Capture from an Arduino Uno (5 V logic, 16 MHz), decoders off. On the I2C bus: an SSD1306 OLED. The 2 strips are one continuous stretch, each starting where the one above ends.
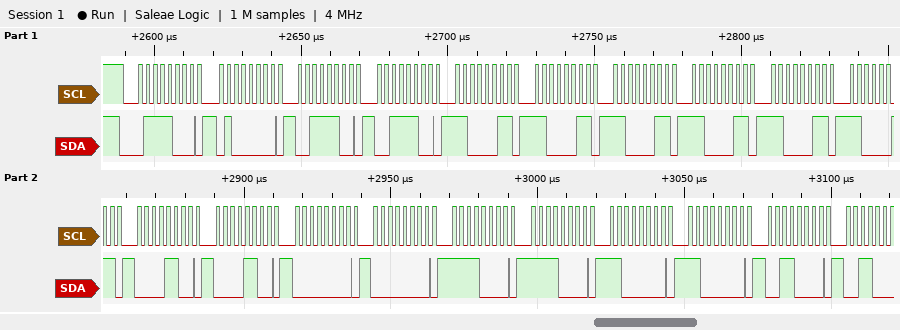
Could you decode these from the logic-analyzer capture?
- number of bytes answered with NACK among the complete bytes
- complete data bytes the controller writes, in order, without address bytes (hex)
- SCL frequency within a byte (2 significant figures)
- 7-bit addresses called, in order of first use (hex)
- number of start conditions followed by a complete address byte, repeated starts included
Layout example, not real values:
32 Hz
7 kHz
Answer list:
0
40 3C 3C C3 C3 C3 C3 C3 C3 0C 0C 00 00 F0 F0 C0 C0 30
400 kHz
0x3C
1
